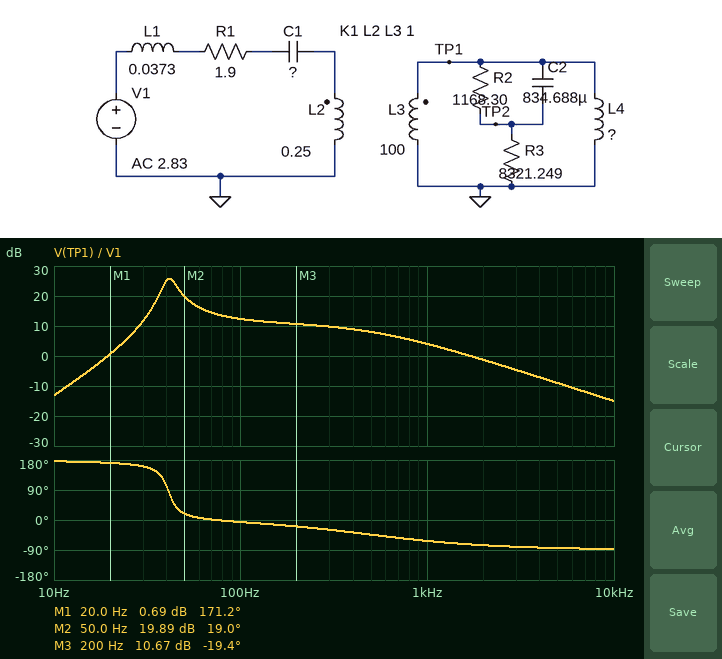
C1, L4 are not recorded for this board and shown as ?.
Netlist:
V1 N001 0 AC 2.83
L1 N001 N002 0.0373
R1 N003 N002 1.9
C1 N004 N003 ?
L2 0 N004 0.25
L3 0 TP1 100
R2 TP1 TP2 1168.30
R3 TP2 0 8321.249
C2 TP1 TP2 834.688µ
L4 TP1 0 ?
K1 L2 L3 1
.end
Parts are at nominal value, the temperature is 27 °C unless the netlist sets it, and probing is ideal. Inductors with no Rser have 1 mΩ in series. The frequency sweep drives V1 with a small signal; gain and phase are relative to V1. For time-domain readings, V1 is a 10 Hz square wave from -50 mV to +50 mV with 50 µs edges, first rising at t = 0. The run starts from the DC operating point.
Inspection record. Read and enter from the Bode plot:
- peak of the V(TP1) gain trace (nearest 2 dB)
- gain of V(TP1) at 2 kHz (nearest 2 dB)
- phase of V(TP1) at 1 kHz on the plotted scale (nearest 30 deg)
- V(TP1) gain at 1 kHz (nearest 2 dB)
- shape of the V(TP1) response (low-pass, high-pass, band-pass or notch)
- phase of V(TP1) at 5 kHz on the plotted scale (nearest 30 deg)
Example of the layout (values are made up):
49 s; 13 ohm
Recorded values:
26 dB; -2 dB; -60 deg; 4 dB; band-pass; -90 deg
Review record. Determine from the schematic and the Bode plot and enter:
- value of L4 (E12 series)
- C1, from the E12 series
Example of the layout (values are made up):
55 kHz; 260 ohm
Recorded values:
3.3 H; 330 µF
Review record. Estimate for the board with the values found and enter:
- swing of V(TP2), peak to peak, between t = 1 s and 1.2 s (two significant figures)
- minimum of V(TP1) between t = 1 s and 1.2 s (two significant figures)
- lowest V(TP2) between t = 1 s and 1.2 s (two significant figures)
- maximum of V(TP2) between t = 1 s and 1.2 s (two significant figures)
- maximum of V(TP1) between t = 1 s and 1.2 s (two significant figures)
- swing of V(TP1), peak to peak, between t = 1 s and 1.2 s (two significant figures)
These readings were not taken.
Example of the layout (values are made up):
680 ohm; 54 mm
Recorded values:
500 mV; -250 mV; -250 mV; 250 mV; 250 mV; 500 mV
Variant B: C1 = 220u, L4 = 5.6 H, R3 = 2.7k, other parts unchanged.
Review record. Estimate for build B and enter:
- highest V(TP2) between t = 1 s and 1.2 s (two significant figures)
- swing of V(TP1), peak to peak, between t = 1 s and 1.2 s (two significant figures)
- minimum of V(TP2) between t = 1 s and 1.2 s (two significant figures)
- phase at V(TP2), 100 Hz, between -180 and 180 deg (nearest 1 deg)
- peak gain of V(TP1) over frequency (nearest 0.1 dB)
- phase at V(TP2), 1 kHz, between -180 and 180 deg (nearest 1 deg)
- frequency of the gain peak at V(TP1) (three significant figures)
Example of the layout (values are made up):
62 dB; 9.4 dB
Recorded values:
410 mV; 820 mV; -410 mV; -34 deg; 25.5 dB; -83 deg; 49.5 Hz
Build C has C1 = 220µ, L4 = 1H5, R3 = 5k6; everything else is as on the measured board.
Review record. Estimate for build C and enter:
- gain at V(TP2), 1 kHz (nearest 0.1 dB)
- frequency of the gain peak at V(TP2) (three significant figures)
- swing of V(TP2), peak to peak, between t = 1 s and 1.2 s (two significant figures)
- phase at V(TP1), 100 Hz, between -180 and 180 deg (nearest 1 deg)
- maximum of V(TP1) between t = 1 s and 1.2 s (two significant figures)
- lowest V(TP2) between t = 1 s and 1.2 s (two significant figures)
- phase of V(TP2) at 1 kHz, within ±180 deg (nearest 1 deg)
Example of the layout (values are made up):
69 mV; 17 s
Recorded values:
0 dB; 53.3 Hz; 350 mV; -2 deg; 180 mV; -180 mV; -56 deg
